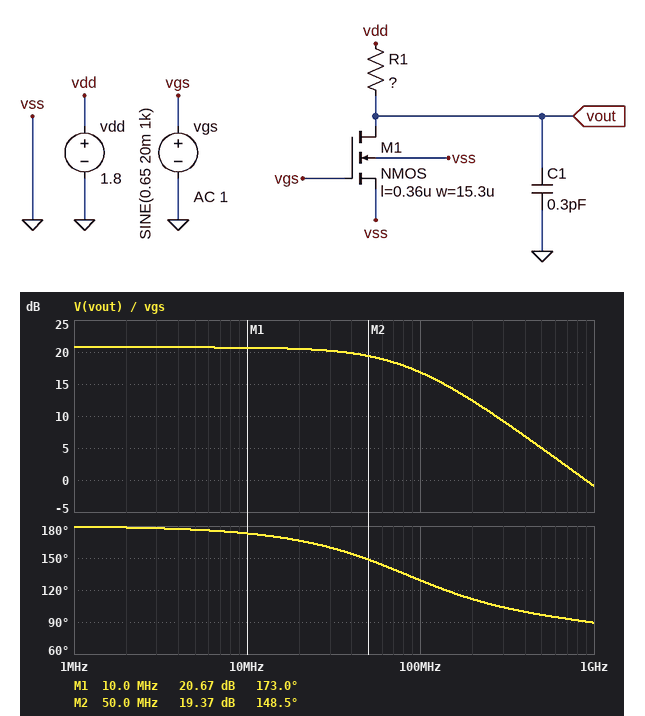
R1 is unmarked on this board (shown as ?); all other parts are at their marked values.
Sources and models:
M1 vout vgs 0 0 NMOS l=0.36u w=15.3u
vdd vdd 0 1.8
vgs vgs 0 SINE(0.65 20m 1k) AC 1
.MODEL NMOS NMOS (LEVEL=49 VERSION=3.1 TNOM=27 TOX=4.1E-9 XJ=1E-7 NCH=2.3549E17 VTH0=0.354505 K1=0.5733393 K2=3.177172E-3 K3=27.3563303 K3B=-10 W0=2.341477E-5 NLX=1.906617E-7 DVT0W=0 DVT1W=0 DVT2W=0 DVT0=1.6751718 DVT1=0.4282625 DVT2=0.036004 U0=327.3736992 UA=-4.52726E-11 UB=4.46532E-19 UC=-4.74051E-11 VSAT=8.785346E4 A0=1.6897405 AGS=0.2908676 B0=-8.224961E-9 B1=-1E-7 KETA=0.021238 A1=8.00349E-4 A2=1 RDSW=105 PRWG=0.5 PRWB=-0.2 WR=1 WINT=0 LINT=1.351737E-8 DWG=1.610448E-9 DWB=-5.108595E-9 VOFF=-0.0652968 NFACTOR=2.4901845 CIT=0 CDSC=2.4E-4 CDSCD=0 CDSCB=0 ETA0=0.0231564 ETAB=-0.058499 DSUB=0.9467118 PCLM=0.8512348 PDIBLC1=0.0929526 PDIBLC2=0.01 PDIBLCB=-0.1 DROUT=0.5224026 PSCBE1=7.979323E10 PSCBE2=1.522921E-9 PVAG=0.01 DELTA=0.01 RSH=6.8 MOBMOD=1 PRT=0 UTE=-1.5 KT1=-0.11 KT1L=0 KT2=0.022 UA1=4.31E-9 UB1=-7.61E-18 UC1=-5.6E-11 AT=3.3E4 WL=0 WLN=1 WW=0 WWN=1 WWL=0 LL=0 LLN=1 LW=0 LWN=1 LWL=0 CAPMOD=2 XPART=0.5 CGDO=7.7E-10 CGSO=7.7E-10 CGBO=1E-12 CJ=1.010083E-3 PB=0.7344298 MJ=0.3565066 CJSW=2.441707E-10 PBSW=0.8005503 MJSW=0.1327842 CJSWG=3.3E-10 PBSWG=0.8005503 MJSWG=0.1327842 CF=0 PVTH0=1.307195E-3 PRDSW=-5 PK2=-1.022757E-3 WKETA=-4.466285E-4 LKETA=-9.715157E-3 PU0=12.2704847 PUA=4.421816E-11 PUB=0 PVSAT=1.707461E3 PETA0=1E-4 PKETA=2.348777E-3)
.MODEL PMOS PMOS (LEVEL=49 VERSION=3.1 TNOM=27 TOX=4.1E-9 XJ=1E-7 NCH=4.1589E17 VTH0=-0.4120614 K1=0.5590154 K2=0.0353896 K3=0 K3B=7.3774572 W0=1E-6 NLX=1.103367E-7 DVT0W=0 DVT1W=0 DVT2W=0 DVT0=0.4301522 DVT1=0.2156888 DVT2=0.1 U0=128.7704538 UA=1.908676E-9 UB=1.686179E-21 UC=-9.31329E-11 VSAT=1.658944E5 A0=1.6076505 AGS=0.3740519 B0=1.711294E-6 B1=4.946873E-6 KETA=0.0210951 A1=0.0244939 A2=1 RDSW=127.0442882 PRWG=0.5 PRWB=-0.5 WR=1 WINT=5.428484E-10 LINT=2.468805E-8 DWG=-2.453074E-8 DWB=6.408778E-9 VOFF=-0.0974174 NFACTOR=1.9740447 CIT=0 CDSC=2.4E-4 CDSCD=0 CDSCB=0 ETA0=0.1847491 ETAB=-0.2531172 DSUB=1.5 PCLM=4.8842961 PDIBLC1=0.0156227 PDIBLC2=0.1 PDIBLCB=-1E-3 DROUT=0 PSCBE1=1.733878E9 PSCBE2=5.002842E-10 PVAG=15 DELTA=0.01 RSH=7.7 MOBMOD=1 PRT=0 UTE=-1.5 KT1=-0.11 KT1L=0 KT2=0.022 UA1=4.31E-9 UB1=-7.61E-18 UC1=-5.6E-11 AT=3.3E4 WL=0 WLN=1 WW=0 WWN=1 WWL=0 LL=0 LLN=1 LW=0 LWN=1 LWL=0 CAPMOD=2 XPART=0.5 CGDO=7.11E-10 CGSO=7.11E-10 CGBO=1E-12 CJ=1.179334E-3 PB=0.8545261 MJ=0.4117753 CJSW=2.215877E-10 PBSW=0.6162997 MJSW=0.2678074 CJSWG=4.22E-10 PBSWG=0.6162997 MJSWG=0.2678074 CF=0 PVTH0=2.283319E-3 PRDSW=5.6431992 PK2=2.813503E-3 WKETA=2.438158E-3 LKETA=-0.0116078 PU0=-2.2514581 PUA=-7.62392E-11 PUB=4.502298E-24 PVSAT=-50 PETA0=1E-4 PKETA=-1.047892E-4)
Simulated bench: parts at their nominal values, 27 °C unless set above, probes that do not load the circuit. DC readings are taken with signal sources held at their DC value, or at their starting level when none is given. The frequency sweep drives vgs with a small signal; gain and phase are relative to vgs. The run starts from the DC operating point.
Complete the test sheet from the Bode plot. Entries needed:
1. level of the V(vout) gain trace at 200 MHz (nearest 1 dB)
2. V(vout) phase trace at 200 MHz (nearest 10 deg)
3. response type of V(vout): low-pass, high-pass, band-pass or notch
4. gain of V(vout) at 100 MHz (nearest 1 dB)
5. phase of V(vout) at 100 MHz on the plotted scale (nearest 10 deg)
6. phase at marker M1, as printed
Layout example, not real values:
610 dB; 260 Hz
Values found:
12 dB; 110 deg; low-pass; 17 dB; 130 deg; 173.0 deg
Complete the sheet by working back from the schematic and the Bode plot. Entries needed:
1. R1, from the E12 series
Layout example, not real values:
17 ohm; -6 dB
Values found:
6.8 kΩ
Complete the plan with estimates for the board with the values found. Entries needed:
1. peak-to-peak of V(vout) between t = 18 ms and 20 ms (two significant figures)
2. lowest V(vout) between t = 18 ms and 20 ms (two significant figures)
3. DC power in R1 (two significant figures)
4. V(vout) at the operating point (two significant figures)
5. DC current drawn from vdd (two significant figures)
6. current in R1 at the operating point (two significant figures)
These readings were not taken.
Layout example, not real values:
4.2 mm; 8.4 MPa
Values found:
430 mV; 570 mV; 150 µW; 800 mV; 150 µA; 150 µA
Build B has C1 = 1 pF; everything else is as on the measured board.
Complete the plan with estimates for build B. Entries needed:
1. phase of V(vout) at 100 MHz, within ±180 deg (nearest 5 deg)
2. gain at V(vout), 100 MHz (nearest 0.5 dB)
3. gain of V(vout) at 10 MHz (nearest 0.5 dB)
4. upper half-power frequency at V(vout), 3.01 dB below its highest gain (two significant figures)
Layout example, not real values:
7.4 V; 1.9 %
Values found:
105 deg; 8.5 dB; 20.0 dB; 26 MHz
